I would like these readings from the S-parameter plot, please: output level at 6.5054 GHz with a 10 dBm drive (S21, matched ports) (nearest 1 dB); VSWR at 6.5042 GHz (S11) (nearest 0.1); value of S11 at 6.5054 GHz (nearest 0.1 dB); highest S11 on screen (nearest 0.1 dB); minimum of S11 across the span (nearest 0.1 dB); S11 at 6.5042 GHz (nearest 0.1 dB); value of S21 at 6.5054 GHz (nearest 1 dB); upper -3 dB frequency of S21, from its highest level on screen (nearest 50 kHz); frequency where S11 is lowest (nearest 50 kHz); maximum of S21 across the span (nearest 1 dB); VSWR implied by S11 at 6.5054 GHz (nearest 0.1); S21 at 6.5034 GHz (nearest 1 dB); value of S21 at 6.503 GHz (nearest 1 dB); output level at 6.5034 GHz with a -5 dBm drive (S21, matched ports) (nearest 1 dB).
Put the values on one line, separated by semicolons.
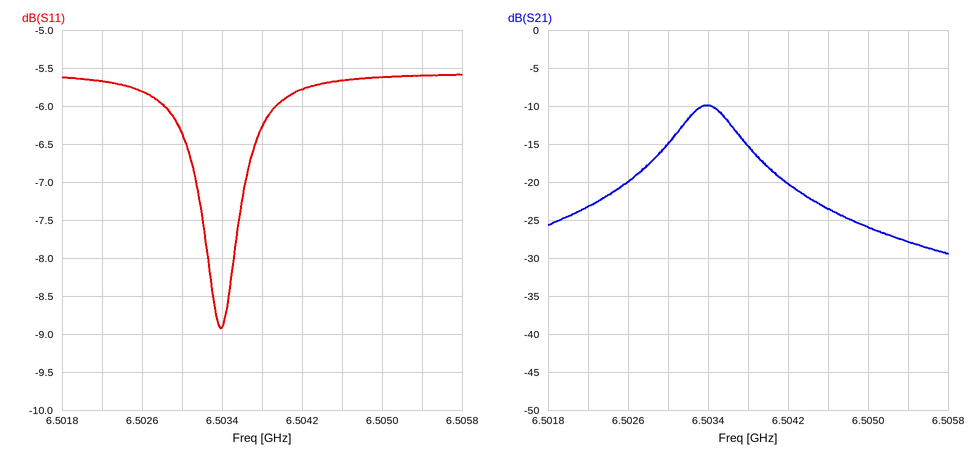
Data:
-18 dBm; 3.1; -5.6 dB; -5.6 dB; -8.9 dB; -5.8 dB; -28 dB; 6.50365 GHz; 6.50340 GHz; -10 dB; 3.2; -10 dB; -15 dB; -15 dBm
